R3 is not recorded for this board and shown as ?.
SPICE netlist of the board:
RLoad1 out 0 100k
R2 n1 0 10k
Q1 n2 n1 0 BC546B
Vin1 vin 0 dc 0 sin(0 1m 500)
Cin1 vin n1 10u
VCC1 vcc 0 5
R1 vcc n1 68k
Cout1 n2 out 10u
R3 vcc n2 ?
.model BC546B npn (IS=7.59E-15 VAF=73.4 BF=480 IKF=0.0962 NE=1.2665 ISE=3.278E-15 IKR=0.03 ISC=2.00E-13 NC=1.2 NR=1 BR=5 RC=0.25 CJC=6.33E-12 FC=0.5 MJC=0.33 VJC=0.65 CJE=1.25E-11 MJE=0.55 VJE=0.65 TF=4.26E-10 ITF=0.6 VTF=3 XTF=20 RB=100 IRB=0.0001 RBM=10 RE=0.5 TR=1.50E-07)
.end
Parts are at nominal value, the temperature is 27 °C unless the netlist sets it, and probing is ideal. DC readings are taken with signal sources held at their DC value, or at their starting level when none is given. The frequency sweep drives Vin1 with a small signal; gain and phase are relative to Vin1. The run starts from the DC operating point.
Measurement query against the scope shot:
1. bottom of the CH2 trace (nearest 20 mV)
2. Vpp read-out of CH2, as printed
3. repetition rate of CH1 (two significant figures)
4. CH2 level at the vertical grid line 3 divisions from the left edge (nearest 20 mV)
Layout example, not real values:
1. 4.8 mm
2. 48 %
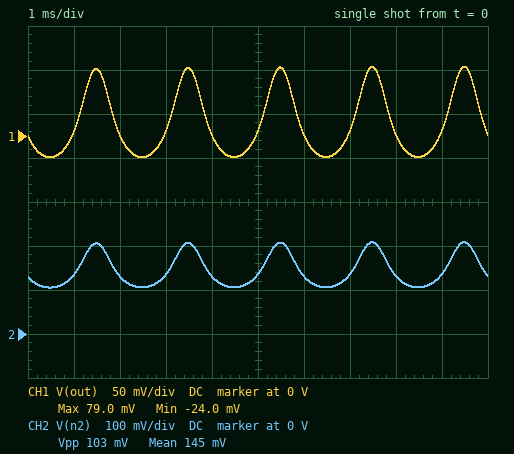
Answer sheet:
1. 100 mV
2. 103 mV
3. 500 Hz
4. 140 mV
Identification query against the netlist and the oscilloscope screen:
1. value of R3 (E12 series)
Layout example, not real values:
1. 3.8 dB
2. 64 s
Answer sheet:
1. 27 kΩ
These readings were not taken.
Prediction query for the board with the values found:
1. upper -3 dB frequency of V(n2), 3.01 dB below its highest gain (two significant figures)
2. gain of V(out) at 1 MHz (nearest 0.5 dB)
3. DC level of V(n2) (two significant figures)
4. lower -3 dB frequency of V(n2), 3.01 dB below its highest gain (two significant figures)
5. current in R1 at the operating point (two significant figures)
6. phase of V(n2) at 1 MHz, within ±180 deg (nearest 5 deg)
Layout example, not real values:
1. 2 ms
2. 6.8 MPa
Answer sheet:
1. 1.1 MHz
2. 28.5 dB
3. 130 mV
4. 35 Hz
5. 64 µA
6. 135 deg
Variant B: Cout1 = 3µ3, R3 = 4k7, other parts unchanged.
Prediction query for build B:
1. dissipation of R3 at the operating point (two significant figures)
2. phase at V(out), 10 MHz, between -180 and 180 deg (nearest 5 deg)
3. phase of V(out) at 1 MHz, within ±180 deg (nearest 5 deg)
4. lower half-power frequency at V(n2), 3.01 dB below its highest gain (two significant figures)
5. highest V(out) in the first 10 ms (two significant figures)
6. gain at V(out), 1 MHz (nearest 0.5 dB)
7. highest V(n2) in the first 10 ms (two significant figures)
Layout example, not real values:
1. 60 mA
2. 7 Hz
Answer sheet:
1. 400 µW
2. 110 deg
3. 165 deg
4. 2.5 Hz
5. 48 mV
6. 33.5 dB
7. 3.7 V
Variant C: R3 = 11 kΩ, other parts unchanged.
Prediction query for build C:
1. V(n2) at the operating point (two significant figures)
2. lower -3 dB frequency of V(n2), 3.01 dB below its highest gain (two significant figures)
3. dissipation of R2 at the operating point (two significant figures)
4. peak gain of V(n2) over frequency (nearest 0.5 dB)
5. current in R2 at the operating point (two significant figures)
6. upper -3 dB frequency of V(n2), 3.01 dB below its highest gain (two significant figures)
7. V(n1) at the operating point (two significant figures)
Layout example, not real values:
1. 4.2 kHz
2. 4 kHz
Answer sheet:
1. 1.9 V
2. 2.5 Hz
3. 40 µW
4. 40.5 dB
5. 63 µA
6. 1.8 MHz
7. 630 mV
